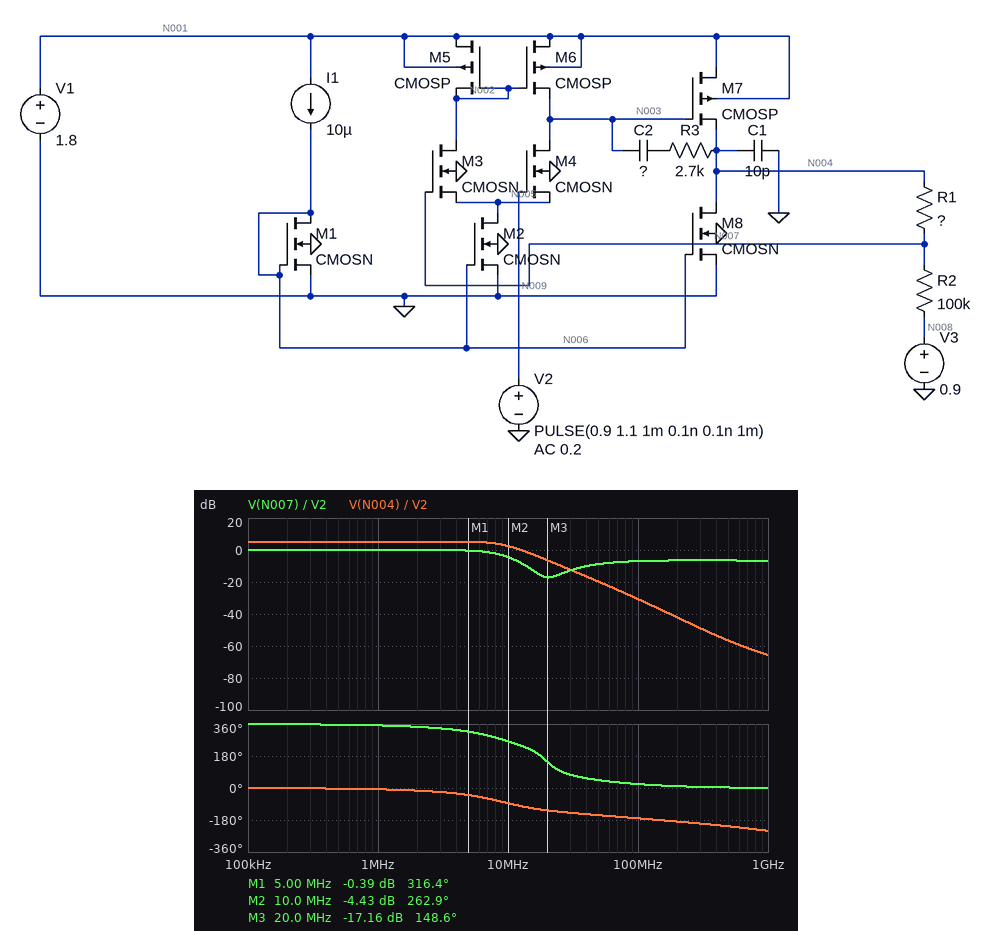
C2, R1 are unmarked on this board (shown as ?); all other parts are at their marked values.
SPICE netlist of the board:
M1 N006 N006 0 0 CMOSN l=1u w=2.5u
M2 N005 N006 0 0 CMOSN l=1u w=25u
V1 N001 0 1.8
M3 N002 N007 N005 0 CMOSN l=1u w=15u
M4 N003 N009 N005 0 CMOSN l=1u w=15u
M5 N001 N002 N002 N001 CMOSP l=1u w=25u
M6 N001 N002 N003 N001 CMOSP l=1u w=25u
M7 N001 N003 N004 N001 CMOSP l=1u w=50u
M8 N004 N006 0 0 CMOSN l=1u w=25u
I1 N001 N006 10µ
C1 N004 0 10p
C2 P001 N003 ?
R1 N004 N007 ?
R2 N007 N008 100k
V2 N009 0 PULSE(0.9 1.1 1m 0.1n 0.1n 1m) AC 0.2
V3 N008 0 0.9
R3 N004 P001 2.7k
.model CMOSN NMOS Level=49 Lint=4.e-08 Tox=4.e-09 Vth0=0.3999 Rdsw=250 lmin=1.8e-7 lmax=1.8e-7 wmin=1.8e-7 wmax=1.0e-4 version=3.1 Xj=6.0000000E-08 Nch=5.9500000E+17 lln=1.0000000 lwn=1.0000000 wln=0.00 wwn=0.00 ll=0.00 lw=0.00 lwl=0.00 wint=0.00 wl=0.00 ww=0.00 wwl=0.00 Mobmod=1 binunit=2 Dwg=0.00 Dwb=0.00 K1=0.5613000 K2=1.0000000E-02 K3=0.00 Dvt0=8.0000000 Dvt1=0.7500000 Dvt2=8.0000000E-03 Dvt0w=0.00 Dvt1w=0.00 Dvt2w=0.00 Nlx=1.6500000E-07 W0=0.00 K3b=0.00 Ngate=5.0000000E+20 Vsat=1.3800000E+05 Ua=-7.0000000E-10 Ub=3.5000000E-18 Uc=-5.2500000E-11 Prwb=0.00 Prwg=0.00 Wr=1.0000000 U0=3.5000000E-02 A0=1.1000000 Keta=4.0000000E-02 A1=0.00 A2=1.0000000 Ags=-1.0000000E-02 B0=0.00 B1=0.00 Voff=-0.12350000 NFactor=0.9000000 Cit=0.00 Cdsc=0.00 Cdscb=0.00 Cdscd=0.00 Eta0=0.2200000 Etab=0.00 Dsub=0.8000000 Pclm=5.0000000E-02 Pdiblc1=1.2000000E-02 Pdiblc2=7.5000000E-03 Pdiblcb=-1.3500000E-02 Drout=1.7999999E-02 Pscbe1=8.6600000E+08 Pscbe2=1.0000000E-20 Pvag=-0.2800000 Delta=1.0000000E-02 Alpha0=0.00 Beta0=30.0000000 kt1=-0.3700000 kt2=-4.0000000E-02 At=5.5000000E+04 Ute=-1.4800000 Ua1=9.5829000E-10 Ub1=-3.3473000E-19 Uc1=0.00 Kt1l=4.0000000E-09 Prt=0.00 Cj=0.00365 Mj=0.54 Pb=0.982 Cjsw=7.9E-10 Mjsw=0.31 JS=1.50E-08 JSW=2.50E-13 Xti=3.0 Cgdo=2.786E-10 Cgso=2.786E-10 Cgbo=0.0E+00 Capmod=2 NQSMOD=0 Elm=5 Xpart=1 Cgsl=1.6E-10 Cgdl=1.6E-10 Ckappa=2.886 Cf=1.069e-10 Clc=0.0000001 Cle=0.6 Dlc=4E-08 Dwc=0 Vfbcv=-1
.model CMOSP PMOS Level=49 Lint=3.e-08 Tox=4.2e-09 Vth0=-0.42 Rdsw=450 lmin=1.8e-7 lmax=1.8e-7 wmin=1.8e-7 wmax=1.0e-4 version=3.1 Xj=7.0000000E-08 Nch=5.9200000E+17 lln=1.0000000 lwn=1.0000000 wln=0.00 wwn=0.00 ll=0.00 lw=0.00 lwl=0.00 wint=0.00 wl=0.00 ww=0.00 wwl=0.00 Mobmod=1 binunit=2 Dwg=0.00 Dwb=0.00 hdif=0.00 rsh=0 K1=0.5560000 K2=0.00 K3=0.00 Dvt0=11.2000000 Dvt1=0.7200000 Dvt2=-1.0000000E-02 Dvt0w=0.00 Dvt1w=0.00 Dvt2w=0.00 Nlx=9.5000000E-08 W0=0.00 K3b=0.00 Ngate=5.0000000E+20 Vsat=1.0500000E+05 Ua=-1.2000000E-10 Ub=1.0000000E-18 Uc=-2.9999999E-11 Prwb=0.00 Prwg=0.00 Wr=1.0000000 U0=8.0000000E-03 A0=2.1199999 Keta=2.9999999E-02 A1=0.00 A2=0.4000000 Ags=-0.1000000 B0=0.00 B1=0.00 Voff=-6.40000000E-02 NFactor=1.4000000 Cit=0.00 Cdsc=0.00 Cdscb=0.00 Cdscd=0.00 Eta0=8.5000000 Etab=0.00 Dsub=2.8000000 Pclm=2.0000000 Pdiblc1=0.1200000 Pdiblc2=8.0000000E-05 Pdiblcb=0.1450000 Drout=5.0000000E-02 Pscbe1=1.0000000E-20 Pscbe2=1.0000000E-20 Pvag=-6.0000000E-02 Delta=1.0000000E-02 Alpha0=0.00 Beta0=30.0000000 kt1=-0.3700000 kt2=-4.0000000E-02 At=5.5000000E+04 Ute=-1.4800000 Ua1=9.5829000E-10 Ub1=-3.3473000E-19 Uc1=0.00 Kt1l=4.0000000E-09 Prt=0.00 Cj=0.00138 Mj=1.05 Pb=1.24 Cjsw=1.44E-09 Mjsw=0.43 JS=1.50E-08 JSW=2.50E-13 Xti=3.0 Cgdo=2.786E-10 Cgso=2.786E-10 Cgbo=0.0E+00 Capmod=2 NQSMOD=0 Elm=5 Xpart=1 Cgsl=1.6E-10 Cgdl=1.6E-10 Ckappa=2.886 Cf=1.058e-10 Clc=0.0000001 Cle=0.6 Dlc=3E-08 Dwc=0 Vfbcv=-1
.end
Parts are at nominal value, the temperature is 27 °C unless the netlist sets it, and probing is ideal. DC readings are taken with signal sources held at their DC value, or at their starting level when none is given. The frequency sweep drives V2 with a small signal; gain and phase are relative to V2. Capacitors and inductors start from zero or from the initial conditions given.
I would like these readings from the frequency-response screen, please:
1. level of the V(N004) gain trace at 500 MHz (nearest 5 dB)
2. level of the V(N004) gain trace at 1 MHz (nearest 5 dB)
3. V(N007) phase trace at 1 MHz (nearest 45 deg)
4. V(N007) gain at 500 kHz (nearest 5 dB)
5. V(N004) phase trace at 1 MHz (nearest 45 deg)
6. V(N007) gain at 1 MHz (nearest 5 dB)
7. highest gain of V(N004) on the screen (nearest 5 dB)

-55 dB
5 dB
360 deg
0 dB
0 deg
0 dB
5 dB
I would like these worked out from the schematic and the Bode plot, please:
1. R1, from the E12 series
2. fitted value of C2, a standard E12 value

82 kΩ
5.6 pF
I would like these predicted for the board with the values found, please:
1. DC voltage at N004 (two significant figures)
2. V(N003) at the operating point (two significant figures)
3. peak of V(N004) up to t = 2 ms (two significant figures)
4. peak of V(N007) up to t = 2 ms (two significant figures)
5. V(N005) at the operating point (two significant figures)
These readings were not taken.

900 mV
1.1 V
1.3 V
1.1 V
250 mV
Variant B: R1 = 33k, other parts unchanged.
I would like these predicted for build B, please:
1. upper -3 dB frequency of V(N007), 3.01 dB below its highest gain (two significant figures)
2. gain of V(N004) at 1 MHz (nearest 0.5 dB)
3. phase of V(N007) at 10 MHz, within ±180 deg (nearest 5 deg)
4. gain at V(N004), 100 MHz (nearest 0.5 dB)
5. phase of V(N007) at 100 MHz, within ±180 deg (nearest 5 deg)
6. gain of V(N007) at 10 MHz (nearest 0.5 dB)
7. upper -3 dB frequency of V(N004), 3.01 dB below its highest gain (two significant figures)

12 MHz
2.5 dB
-75 deg
-29.0 dB
40 deg
-1.5 dB
13 MHz
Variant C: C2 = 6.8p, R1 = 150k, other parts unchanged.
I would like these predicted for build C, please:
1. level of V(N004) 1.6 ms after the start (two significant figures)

1.4 V
